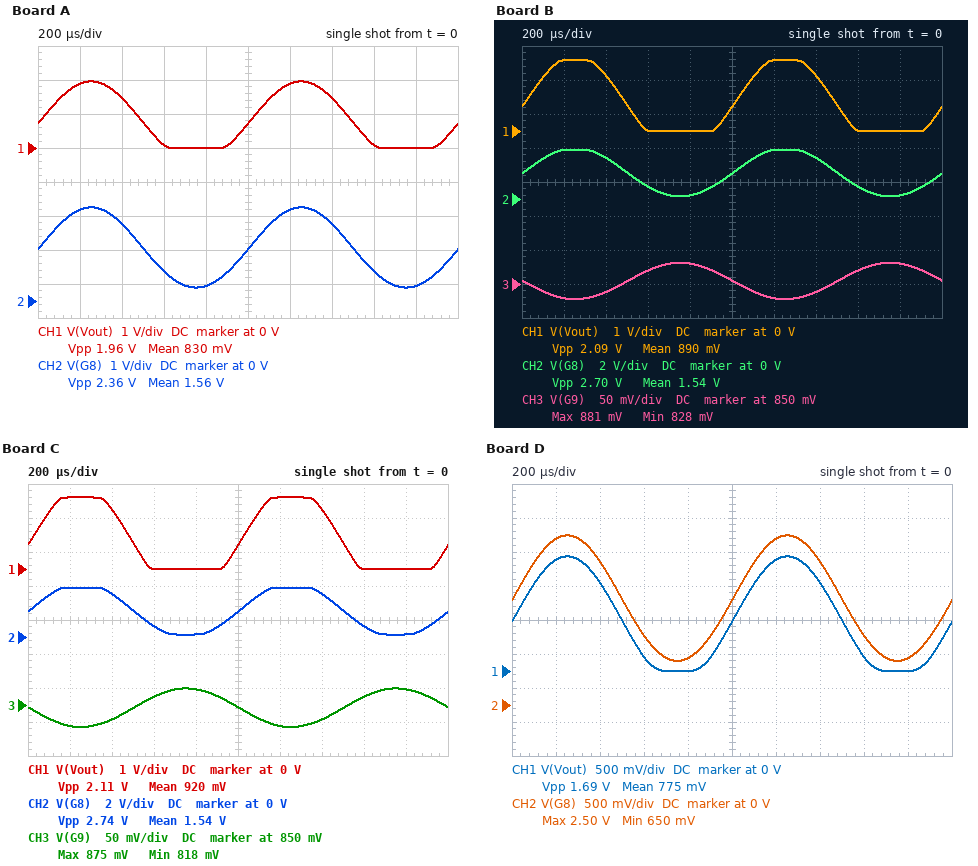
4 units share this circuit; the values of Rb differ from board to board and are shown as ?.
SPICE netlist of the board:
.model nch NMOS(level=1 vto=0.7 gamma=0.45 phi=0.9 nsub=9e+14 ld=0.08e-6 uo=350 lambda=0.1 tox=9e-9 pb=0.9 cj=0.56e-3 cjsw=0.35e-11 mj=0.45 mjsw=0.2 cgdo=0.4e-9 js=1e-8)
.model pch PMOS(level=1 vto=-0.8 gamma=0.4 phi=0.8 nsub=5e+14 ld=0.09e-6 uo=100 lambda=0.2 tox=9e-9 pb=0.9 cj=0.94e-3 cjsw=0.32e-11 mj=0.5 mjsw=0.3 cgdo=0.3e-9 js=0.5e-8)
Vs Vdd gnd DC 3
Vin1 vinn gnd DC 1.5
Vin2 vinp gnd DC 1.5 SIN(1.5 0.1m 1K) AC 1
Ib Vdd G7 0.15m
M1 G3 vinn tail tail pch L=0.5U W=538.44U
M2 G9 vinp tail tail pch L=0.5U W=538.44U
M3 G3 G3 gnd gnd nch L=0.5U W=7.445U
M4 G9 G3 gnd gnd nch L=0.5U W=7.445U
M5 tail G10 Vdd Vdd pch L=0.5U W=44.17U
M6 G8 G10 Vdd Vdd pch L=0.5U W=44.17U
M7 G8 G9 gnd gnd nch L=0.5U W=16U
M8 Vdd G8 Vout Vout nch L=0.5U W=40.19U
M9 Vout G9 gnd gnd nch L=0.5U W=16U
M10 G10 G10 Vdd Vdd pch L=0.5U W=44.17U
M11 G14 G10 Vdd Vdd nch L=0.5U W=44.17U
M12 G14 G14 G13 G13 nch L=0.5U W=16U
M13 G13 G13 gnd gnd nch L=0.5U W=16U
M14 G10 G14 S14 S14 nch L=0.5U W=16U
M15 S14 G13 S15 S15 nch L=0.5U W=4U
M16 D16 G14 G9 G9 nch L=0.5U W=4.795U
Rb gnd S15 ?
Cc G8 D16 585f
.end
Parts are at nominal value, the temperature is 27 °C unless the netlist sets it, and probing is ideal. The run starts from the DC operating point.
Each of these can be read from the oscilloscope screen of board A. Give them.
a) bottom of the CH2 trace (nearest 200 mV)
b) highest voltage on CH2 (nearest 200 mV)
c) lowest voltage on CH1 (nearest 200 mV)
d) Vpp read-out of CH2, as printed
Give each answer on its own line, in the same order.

400 mV
2.8 V
0 V
2.36 V
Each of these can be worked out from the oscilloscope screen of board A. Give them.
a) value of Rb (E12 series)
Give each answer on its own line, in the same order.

1.5 kΩ
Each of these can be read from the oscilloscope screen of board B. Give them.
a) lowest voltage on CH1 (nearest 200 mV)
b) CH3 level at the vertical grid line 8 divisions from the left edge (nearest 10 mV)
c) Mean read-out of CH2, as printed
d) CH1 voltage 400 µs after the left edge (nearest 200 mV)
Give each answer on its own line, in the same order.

0 V
870 mV
1.54 V
1.6 V
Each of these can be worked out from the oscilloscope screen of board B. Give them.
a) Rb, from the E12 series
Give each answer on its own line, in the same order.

2.2 kΩ
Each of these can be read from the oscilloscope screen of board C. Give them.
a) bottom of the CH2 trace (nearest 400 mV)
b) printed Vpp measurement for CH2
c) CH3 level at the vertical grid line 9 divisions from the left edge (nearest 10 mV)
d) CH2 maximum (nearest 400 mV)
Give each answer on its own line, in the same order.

0 V
2.74 V
870 mV
2.8 V
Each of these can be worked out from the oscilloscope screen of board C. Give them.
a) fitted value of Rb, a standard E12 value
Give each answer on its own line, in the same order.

2.7 kΩ
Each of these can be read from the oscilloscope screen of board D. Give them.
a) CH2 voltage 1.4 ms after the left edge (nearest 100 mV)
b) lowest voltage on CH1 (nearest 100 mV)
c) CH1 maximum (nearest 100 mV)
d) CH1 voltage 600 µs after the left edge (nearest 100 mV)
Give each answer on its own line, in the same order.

2.1 V
0 V
1.7 V
200 mV
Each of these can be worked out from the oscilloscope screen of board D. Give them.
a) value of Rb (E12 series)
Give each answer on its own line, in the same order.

820 Ω
